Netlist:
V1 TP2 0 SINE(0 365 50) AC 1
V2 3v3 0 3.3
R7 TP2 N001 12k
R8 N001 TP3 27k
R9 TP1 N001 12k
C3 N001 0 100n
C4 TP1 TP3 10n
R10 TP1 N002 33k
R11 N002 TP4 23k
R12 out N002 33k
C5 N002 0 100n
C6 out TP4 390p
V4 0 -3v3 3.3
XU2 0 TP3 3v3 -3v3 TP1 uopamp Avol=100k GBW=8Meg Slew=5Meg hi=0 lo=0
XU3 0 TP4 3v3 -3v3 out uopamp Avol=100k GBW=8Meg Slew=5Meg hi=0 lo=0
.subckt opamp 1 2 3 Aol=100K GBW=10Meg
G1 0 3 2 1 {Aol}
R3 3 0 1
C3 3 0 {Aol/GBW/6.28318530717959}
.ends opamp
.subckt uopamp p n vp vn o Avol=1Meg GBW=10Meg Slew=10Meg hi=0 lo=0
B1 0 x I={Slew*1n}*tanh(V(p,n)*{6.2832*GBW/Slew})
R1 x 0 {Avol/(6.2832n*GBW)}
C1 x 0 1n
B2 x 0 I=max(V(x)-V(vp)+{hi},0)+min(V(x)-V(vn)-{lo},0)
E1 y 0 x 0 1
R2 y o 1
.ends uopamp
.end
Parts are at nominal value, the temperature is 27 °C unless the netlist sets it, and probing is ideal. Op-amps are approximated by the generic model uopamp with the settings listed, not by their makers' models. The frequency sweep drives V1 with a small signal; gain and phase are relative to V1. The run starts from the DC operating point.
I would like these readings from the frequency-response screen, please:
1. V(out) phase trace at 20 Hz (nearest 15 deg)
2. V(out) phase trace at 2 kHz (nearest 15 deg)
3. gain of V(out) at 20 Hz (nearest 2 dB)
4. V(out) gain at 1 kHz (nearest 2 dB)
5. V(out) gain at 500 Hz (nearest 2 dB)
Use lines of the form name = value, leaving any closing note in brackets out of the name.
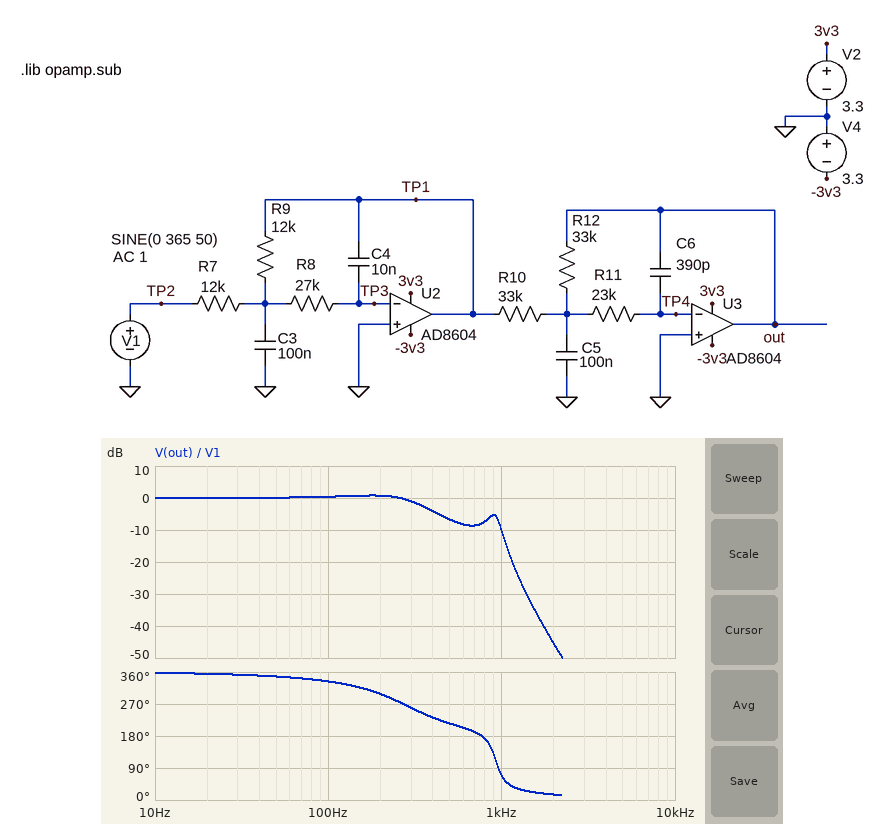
V(out) phase trace at 20 Hz = 360 deg
V(out) phase trace at 2 kHz = 15 deg
gain of V(out) at 20 Hz = 0 dB
V(out) gain at 1 kHz = -10 dB
V(out) gain at 500 Hz = -6 dB
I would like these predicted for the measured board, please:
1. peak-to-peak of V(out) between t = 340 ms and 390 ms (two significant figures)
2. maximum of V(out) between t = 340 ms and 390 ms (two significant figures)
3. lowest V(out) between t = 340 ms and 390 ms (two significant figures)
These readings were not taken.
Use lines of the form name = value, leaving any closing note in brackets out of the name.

peak-to-peak of V(out) between t = 340 ms and 390 ms = 6.6 V
maximum of V(out) between t = 340 ms and 390 ms = 3.3 V
lowest V(out) between t = 340 ms and 390 ms = -3.3 V
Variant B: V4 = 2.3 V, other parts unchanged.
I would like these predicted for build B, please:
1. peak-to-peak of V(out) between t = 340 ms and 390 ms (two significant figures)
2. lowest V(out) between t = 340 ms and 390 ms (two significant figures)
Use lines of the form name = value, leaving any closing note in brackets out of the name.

peak-to-peak of V(out) between t = 340 ms and 390 ms = 5.6 V
lowest V(out) between t = 340 ms and 390 ms = -2.3 V
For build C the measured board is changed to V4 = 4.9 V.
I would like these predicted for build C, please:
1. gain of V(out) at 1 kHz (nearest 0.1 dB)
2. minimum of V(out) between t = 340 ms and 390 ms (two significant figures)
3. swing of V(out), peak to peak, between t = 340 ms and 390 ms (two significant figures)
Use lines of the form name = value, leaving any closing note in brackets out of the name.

gain of V(out) at 1 kHz = -10.2 dB
minimum of V(out) between t = 340 ms and 390 ms = -4.9 V
swing of V(out), peak to peak, between t = 340 ms and 390 ms = 8.2 V
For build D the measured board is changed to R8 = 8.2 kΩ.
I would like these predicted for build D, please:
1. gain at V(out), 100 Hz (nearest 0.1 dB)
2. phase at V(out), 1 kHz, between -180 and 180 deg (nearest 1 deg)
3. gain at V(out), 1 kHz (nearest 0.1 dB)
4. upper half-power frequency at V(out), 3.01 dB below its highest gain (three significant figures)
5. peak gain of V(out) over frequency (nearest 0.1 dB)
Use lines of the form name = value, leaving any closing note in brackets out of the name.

gain at V(out), 100 Hz = 0.3 dB
phase at V(out), 1 kHz, between -180 and 180 deg = 80 deg
gain at V(out), 1 kHz = 1.1 dB
upper half-power frequency at V(out), 3.01 dB below its highest gain = 972 Hz
peak gain of V(out) over frequency = 6.2 dB
